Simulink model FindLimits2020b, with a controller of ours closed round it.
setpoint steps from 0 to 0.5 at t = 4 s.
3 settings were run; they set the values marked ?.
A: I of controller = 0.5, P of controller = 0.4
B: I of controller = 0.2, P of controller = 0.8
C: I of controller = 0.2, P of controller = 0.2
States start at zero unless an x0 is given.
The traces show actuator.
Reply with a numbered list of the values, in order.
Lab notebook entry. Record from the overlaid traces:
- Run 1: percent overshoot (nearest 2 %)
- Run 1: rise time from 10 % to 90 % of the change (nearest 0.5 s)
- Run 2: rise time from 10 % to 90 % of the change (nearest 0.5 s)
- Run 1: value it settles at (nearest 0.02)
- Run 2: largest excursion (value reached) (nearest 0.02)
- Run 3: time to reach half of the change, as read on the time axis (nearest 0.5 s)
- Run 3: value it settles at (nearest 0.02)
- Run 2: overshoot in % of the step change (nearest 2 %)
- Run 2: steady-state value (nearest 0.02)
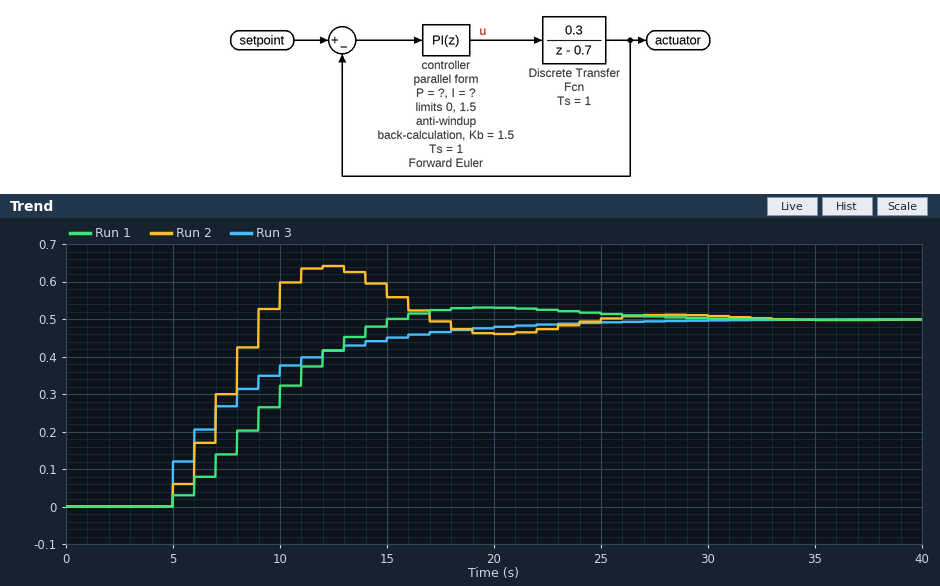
1. 6 %
2. 7.0 s
3. 4.0 s
4. 0.50
5. 0.64
6. 7.0 s
7. 0.50
8. 28 %
9. 0.50
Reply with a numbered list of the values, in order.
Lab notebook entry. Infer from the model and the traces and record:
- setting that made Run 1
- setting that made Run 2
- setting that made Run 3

1. C
2. A
3. B
